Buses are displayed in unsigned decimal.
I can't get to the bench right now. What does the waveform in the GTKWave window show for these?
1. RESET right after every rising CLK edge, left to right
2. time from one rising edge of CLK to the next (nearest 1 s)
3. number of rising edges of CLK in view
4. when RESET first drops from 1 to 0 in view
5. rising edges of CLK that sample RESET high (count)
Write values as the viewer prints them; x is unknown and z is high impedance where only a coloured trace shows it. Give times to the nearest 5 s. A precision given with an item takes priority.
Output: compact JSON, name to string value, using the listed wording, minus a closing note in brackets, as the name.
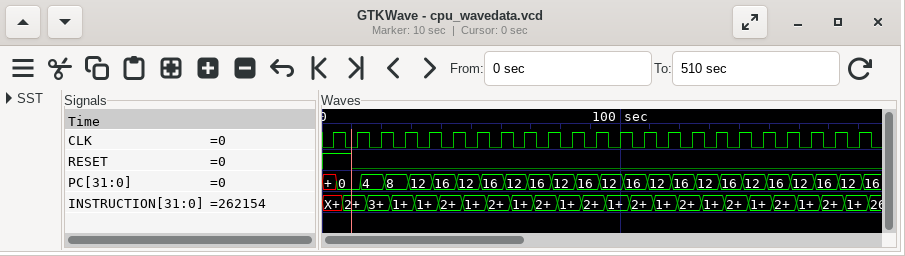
{"RESET right after every rising CLK edge, left to right": "1 0 0 0 0 0 0 0 0 0 0 0 0 0 0 0 0 0 0 0 0 0 0", "time from one rising edge of CLK to the next": "8 s", "number of rising edges of CLK in view": "23", "when RESET first drops from 1 to 0 in view": "10 s", "rising edges of CLK that sample RESET high": "1"}
